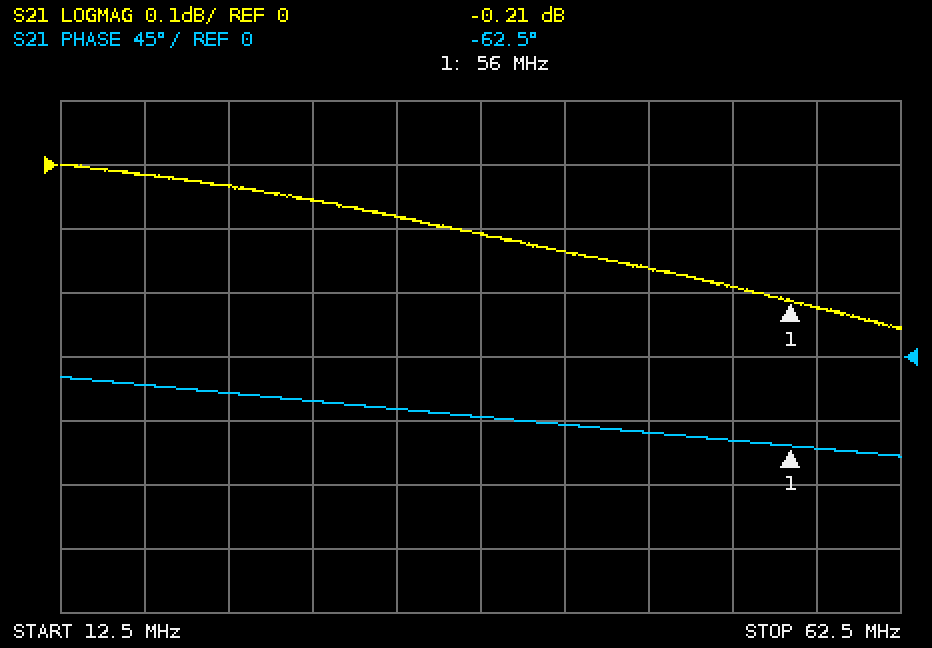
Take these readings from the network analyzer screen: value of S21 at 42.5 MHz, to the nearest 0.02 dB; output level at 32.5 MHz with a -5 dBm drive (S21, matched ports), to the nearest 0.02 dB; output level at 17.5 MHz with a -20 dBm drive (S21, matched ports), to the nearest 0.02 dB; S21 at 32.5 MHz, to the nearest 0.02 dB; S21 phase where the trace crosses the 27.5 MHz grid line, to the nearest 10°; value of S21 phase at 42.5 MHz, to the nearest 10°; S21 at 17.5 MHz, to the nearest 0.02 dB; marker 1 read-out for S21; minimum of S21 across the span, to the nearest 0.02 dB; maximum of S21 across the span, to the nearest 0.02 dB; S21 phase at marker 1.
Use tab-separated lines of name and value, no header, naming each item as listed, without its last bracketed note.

value of S21 at 42.5 MHz, to the nearest 0.02 dB	-0.14 dB
output level at 32.5 MHz with a -5 dBm drive (S21, matched ports), to the nearest 0.02 dB	-5.08 dBm
output level at 17.5 MHz with a -20 dBm drive (S21, matched ports), to the nearest 0.02 dB	-20.02 dBm
S21 at 32.5 MHz, to the nearest 0.02 dB	-0.08 dB
S21 phase where the trace crosses the 27.5 MHz grid line, to the nearest 10°	-30°
value of S21 phase at 42.5 MHz, to the nearest 10°	-50°
S21 at 17.5 MHz, to the nearest 0.02 dB	-0.02 dB
marker 1 read-out for S21	-0.21 dB
minimum of S21 across the span, to the nearest 0.02 dB	-0.26 dB
maximum of S21 across the span, to the nearest 0.02 dB	0.00 dB
S21 phase at marker 1	-62.5°
